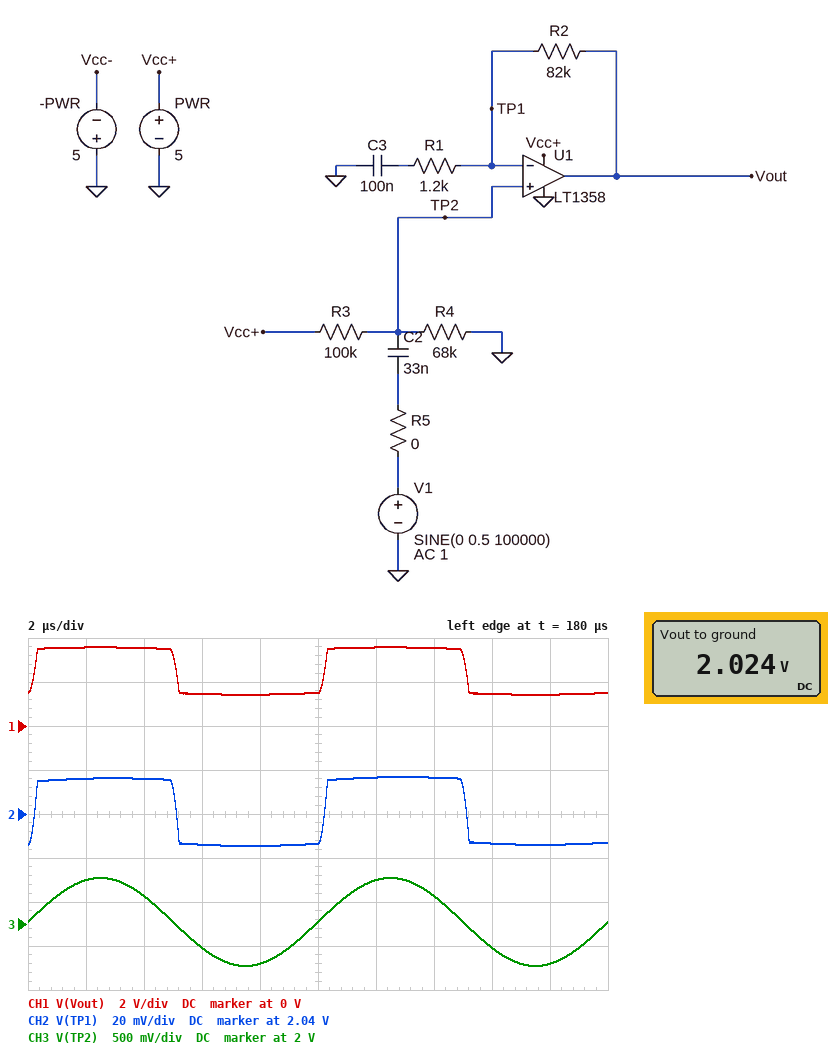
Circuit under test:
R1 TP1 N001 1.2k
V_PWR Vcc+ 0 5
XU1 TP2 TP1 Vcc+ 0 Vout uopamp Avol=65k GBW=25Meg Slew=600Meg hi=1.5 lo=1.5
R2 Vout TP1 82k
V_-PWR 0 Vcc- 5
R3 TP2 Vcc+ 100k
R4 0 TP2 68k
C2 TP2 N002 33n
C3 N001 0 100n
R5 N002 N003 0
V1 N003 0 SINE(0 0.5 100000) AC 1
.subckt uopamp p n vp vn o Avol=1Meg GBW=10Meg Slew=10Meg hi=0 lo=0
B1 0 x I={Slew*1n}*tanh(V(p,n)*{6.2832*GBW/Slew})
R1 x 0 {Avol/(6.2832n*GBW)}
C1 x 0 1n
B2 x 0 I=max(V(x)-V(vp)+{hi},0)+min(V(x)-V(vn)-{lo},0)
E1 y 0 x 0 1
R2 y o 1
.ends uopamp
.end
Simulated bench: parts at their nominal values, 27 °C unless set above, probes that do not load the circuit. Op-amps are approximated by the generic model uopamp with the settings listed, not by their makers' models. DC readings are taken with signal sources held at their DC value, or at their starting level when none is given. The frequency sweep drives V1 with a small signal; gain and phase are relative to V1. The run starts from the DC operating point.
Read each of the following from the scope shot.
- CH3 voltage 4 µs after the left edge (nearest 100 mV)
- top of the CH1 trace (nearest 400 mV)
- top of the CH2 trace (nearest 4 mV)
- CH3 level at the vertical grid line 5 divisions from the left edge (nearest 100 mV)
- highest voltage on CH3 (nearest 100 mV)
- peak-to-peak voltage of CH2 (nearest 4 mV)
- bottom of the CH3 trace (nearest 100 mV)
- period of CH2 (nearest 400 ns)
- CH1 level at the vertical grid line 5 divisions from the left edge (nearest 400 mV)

2.3 V
3.6 V
2.056 V
2.0 V
2.5 V
32 mV
1.5 V
10.0 µs
1.6 V
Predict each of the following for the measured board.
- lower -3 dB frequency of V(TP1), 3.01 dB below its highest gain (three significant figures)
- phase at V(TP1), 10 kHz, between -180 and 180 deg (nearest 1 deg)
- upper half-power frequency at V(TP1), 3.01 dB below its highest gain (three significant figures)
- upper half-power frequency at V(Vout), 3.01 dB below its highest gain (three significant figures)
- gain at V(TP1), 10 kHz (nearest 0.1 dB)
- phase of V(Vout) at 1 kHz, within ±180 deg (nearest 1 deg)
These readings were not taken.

120 Hz
-1 deg
360 kHz
362 kHz
0 dB
59 deg
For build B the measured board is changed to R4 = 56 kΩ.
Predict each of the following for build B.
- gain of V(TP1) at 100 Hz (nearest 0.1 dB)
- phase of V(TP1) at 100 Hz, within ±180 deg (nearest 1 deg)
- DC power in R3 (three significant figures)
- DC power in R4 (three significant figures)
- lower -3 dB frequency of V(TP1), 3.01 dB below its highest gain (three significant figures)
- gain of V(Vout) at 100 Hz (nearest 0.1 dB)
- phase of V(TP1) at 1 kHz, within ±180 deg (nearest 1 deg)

-4.5 dB
53 deg
103 µW
57.5 µW
135 Hz
10.0 dB
8 deg
